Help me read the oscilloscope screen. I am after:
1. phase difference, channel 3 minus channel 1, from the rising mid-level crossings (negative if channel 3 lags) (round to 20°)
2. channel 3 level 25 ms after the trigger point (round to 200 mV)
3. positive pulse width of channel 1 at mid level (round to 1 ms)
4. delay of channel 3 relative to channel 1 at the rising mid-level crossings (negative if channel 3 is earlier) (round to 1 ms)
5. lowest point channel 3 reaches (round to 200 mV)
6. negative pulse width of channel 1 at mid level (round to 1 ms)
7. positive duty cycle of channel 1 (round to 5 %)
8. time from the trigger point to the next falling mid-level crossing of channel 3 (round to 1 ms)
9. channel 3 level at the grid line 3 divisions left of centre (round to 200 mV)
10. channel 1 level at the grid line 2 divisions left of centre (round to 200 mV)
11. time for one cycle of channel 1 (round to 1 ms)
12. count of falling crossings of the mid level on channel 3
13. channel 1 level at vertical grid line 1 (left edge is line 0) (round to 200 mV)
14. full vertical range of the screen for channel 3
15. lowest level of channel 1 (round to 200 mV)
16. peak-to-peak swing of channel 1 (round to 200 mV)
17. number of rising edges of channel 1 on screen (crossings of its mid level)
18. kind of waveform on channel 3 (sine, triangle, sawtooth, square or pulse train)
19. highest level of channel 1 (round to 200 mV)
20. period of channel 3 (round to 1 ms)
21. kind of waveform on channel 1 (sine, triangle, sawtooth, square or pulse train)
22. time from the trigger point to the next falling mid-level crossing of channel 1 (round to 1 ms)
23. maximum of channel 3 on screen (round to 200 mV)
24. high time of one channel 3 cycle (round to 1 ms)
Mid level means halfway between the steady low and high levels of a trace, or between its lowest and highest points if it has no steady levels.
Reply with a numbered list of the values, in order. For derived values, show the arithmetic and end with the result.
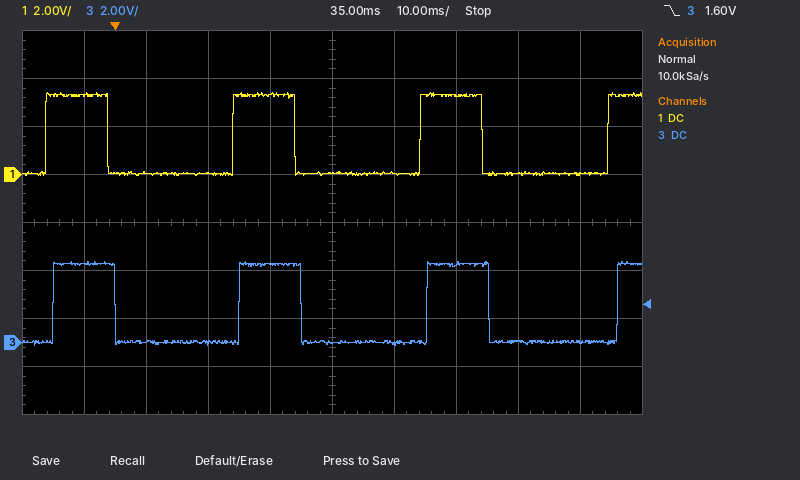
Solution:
1. −360° × (+1 ms) / 30 ms ≈ -12.0°, so -20° to the nearest 20°
2. 3.2 V
3. 10 ms
4. +1 ms
5. -200 mV
6. 20 ms
7. 10 ms / 30 ms ≈ 33.3 %, so 35 % to the nearest 5 %
8. 30 ms
9. 0.0 V
10. 0.0 V
11. 30 ms
12. 3
13. 3.4 V
14. 16 V
15. 0.0 V
16. 3.4 V − (0.0 V) = 3.4 V
17. 4
18. pulse train
19. 3.4 V
20. 30 ms
21. pulse train
22. 29 ms
23. 3.4 V
24. 10 ms
